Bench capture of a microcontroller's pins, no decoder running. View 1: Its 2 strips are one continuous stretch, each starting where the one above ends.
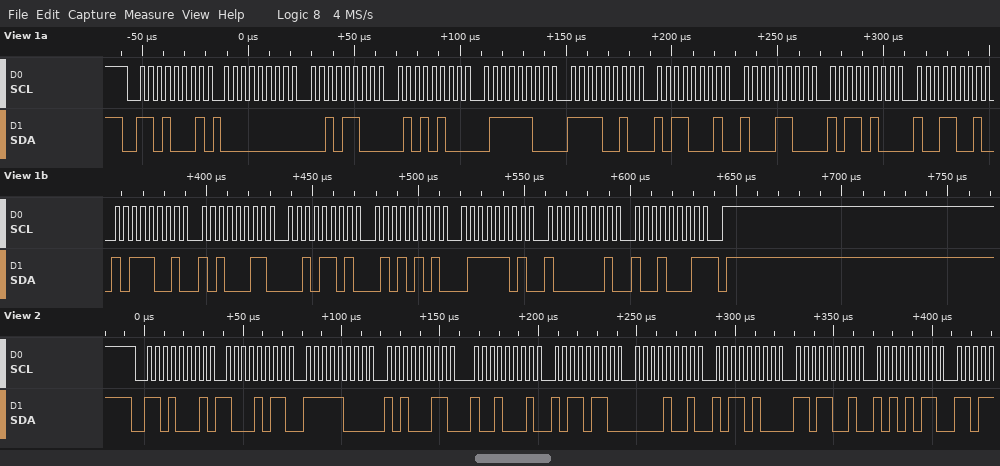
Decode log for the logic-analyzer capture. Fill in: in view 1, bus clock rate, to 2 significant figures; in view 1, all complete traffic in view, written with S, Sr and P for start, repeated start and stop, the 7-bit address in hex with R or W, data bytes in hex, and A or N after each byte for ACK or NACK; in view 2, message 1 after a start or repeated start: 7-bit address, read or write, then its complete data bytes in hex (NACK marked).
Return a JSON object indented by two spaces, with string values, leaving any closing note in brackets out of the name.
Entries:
{
  "in view 1, bus clock rate, to 2 significant figures": "250 kHz",
  "in view 1, all complete traffic in view, written with S, Sr and P for start, repeated start and stop, the 7-bit address in hex with R or W, data bytes in hex, and A or N after each byte for ACK or NACK": "S 68R A 00 A 2C A 54 A 7C A F2 A B1 A 8C A B4 A 99 A B9 A A3 A 2D A 55 A 7D A 81 A 91 N P",
  "in view 2, message 1 after a start or repeated start: 7-bit address, read or write, then its complete data bytes in hex": "0x68 read: 8B F8 A3 91 B6 09 B4 D9 AB"
}
